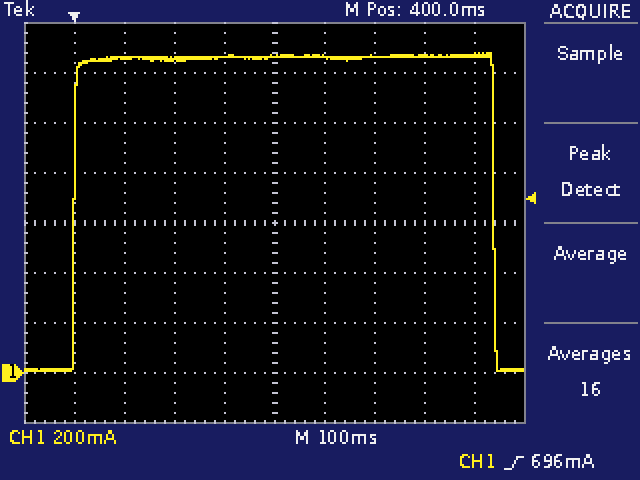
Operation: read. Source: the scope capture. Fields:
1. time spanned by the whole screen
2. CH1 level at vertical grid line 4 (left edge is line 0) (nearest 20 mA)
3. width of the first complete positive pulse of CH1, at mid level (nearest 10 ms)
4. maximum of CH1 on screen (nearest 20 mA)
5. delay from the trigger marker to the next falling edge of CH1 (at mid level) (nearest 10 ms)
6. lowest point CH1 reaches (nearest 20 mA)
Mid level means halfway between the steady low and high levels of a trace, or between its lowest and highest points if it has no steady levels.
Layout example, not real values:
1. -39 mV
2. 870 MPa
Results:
1. 1 s
2. 1.26 A
3. 840 ms
4. 1.28 A
5. 840 ms
6. 0 mA
